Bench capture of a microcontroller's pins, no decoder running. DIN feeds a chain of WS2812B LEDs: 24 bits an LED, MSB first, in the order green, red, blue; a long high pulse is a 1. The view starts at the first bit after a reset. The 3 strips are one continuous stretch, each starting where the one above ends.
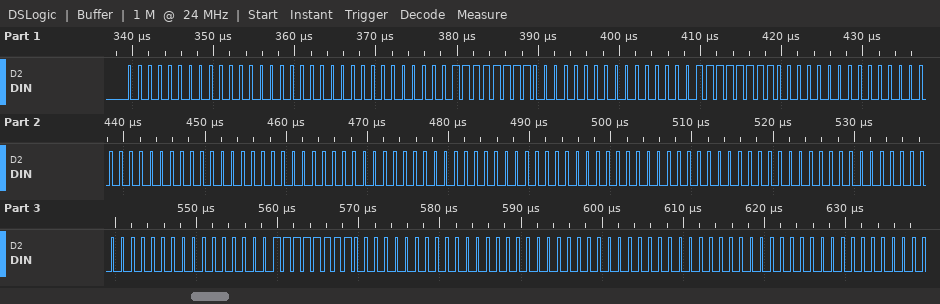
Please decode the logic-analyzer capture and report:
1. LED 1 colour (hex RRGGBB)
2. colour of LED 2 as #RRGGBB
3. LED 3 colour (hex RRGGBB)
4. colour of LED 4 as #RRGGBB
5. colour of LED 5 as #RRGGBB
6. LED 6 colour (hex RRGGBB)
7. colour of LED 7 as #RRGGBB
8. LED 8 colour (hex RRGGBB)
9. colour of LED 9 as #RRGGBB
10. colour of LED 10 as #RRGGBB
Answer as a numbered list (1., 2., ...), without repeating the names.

1. #000000
2. #FF0000
3. #FF0000
4. #000000
5. #000000
6. #000000
7. #000000
8. #FF0000
9. #000000
10. #000000
